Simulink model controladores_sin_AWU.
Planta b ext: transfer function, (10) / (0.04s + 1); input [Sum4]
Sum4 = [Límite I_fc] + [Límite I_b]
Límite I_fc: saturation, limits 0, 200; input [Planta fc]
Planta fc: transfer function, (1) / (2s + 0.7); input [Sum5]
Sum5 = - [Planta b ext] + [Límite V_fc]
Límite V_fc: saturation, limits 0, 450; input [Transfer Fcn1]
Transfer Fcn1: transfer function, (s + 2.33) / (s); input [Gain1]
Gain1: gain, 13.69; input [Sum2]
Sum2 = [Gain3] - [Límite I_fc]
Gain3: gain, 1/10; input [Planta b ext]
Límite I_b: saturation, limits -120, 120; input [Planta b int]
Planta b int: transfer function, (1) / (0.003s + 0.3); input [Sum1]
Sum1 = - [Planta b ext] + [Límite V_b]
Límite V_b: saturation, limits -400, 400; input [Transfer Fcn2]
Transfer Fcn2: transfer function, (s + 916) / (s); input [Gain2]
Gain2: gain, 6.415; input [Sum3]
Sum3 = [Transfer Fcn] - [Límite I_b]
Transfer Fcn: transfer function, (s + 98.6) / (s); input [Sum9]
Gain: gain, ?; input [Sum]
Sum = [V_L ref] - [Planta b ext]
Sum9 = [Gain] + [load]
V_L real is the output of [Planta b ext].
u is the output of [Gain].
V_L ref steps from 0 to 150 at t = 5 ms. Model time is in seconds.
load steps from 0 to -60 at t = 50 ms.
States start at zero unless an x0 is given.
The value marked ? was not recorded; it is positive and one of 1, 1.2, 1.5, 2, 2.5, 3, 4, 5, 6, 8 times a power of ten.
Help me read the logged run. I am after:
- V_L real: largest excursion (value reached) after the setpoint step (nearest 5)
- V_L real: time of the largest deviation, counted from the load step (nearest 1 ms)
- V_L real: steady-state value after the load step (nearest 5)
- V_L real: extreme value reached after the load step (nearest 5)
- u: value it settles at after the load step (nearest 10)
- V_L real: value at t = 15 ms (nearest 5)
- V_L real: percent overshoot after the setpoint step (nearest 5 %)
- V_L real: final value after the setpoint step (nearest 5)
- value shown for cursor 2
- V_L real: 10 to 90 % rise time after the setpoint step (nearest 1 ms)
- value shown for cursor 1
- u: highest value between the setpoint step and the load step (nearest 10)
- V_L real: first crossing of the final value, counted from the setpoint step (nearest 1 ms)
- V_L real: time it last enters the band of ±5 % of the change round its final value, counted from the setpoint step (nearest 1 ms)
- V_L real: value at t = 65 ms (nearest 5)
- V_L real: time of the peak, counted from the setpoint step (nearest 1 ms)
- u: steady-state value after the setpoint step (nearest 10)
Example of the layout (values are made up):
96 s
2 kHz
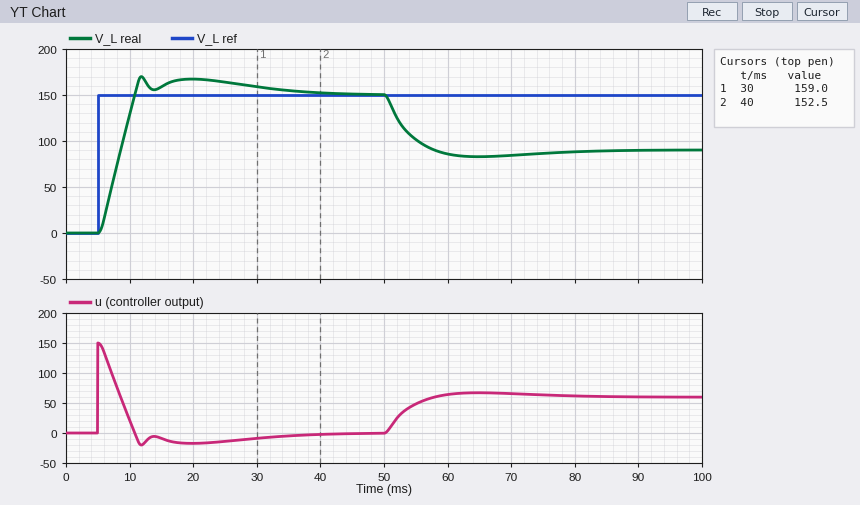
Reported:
170
15 ms
90
85
60
160
15 %
150
152.5
4 ms
159.0
150
6 ms
26 ms
85
7 ms
0
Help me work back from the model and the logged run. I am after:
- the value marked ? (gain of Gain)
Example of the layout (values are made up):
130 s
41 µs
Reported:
1
